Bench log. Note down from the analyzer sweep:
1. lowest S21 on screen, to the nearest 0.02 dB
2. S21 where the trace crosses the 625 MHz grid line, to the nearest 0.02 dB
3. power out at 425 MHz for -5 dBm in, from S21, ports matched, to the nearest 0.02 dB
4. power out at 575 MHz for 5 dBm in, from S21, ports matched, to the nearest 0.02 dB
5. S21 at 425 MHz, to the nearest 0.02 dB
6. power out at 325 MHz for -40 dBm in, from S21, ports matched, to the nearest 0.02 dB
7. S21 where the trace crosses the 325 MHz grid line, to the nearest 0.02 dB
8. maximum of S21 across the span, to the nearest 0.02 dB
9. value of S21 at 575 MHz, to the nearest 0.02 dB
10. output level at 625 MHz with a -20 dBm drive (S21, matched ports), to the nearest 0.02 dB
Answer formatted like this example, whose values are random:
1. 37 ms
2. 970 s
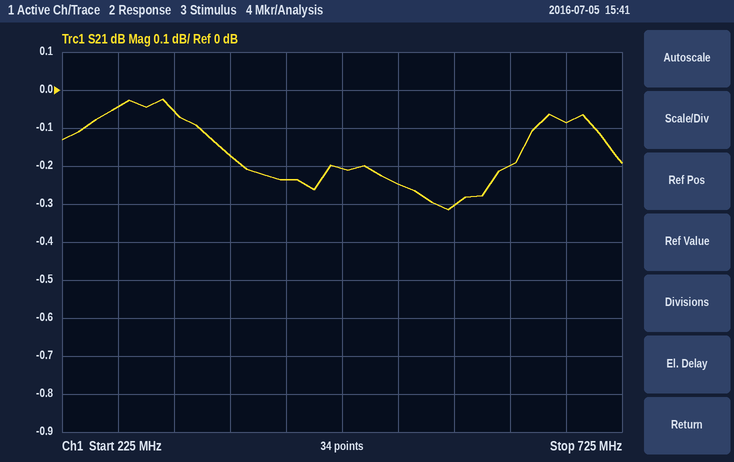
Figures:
1. -0.32 dB
2. -0.20 dB
3. -5.24 dBm
4. 4.70 dBm
5. -0.24 dB
6. -40.06 dBm
7. -0.06 dB
8. -0.02 dB
9. -0.30 dB
10. -20.20 dBm
